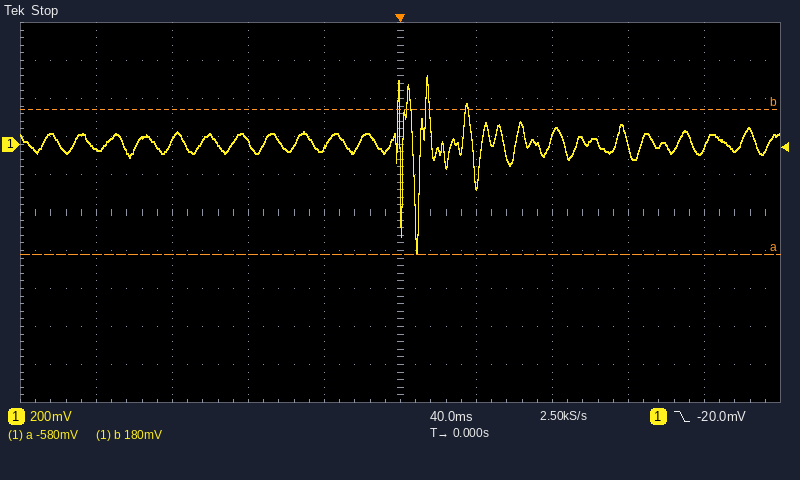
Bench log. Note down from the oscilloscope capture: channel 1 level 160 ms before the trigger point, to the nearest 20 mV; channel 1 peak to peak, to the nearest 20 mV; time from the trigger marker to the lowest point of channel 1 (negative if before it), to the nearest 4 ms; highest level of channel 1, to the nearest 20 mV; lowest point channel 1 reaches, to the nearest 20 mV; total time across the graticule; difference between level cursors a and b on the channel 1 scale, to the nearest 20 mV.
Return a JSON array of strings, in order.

["-20 mV", "940 mV", "+8 ms", "360 mV", "-580 mV", "400 ms", "760 mV"]
